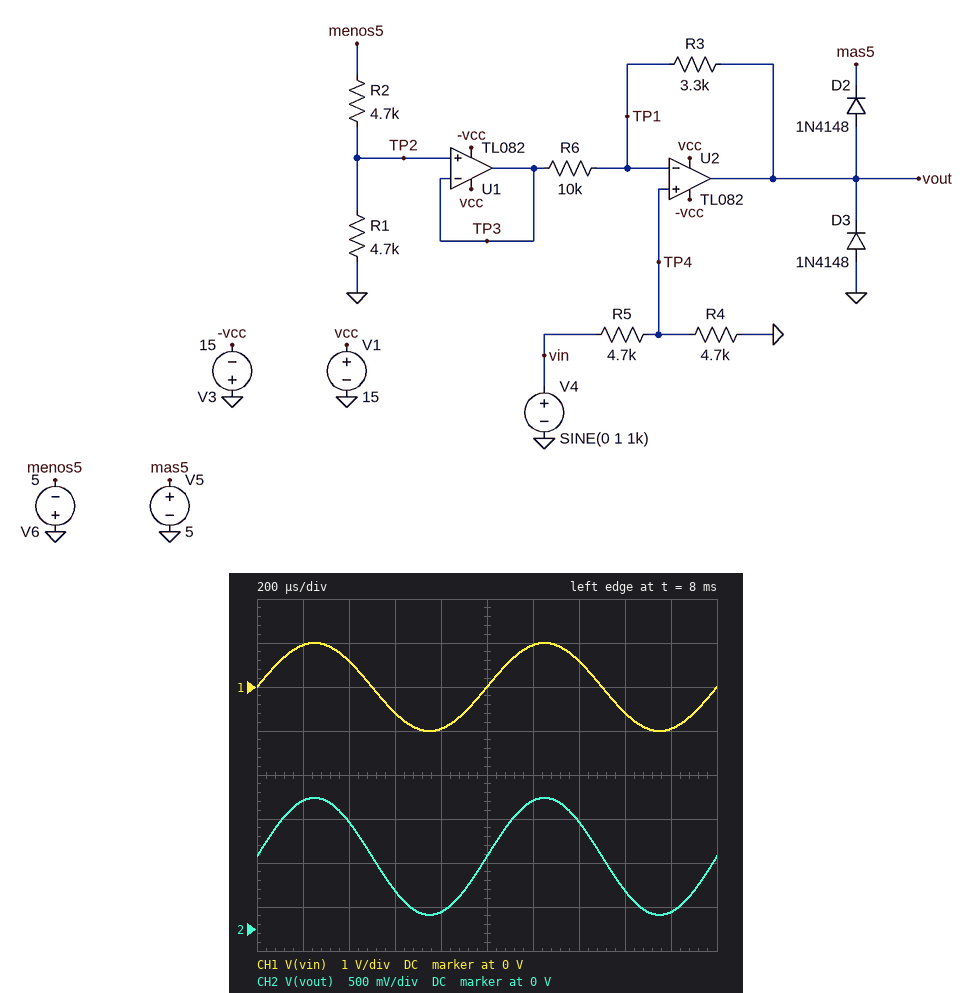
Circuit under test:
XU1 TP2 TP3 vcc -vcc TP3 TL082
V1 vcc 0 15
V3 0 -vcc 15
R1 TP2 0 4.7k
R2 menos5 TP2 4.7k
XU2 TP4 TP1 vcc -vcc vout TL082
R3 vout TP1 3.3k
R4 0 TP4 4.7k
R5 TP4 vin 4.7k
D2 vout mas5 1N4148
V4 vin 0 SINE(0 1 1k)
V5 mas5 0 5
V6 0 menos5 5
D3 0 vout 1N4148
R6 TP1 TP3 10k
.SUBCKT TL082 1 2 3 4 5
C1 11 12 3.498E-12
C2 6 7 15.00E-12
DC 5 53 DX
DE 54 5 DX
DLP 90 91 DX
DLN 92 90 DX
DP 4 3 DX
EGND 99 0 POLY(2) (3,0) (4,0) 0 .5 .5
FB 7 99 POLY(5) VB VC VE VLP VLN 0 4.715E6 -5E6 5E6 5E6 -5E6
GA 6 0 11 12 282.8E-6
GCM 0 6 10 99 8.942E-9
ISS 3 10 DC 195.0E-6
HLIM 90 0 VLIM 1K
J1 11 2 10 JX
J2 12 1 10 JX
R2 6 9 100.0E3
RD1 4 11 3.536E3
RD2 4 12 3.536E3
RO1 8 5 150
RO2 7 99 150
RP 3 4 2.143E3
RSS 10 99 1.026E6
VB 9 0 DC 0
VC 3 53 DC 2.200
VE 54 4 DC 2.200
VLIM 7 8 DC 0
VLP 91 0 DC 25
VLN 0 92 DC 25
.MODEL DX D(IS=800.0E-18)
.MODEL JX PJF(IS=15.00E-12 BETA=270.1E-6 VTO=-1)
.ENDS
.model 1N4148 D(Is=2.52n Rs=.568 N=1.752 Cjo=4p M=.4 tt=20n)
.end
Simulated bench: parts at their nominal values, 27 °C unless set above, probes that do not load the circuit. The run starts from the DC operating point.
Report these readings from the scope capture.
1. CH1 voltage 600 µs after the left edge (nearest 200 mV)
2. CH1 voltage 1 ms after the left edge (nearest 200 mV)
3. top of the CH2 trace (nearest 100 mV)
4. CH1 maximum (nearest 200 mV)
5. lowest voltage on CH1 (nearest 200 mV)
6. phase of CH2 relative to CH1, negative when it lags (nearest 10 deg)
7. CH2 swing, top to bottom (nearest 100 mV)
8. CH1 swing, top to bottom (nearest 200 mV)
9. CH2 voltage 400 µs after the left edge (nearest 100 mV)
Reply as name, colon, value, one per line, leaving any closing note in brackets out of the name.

CH1 voltage 600 µs after the left edge: -600 mV
CH1 voltage 1 ms after the left edge: 0 V
top of the CH2 trace: 1.5 V
CH1 maximum: 1.0 V
lowest voltage on CH1: -1.0 V
phase of CH2 relative to CH1, negative when it lags: 0 deg
CH2 swing, top to bottom: 1.3 V
CH1 swing, top to bottom: 2.0 V
CH2 voltage 400 µs after the left edge: 1.2 V
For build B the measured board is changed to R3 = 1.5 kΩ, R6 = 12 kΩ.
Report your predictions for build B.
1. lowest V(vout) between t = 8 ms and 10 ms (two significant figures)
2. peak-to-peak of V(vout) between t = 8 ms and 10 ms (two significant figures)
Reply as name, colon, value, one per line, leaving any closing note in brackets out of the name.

lowest V(vout) between t = 8 ms and 10 ms: -250 mV
peak-to-peak of V(vout) between t = 8 ms and 10 ms: 1.1 V
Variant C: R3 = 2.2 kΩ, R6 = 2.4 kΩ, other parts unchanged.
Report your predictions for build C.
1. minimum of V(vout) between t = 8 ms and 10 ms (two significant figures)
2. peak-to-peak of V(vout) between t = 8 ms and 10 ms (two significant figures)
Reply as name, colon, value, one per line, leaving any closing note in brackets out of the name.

minimum of V(vout) between t = 8 ms and 10 ms: 1.3 V
peak-to-peak of V(vout) between t = 8 ms and 10 ms: 1.9 V
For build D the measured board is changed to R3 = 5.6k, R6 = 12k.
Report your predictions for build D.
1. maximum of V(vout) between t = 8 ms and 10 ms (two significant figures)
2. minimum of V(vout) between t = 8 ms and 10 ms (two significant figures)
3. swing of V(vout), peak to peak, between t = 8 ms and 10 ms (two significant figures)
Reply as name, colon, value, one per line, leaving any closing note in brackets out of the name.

maximum of V(vout) between t = 8 ms and 10 ms: 1.9 V
minimum of V(vout) between t = 8 ms and 10 ms: 430 mV
swing of V(vout), peak to peak, between t = 8 ms and 10 ms: 1.5 V
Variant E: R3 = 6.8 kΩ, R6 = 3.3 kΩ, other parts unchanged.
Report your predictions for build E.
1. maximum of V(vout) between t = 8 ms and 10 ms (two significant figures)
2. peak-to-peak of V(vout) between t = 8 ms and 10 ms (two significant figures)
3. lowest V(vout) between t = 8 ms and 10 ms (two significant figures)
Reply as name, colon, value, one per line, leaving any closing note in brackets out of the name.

maximum of V(vout) between t = 8 ms and 10 ms: 5.7 V
peak-to-peak of V(vout) between t = 8 ms and 10 ms: 2.1 V
lowest V(vout) between t = 8 ms and 10 ms: 3.6 V
